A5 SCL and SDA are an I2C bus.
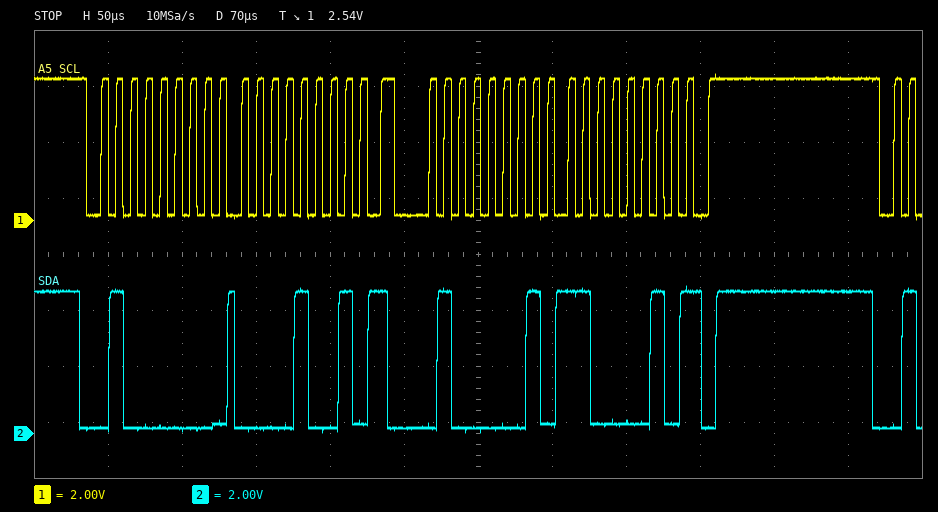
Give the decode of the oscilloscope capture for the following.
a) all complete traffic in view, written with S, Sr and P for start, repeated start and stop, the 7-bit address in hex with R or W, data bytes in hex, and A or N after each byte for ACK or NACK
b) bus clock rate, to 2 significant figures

S 20W A 09 A Sr 20R A C2 N P
100 kHz
